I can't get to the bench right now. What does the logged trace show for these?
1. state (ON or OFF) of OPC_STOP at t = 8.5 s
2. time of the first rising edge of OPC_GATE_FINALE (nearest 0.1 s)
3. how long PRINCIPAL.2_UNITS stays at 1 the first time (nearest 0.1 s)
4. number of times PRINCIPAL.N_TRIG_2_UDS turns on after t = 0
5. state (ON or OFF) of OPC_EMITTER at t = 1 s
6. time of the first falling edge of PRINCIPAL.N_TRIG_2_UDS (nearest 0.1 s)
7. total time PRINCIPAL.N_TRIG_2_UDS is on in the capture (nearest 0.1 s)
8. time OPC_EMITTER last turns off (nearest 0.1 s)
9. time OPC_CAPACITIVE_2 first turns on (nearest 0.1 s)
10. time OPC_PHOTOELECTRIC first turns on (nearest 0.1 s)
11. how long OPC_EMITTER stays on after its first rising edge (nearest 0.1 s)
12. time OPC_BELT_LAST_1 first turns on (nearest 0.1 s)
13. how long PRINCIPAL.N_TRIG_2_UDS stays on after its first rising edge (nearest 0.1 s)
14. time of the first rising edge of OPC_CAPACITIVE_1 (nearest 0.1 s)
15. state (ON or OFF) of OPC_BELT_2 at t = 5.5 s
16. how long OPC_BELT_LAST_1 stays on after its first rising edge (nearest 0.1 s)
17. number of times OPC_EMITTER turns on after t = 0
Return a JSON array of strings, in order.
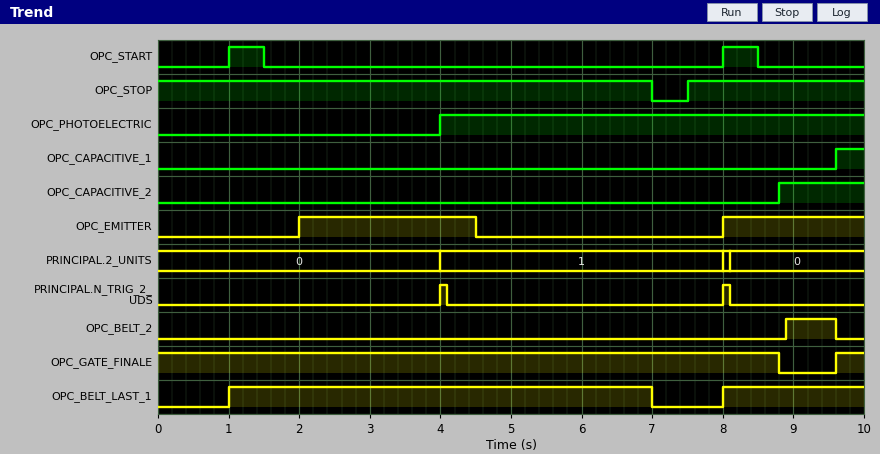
["ON", "9.6 s", "4.0 s", "2", "OFF", "4.1 s", "0.2 s", "4.5 s", "8.8 s", "4.0 s", "2.5 s", "1.0 s", "0.1 s", "9.6 s", "OFF", "6.0 s", "2"]
